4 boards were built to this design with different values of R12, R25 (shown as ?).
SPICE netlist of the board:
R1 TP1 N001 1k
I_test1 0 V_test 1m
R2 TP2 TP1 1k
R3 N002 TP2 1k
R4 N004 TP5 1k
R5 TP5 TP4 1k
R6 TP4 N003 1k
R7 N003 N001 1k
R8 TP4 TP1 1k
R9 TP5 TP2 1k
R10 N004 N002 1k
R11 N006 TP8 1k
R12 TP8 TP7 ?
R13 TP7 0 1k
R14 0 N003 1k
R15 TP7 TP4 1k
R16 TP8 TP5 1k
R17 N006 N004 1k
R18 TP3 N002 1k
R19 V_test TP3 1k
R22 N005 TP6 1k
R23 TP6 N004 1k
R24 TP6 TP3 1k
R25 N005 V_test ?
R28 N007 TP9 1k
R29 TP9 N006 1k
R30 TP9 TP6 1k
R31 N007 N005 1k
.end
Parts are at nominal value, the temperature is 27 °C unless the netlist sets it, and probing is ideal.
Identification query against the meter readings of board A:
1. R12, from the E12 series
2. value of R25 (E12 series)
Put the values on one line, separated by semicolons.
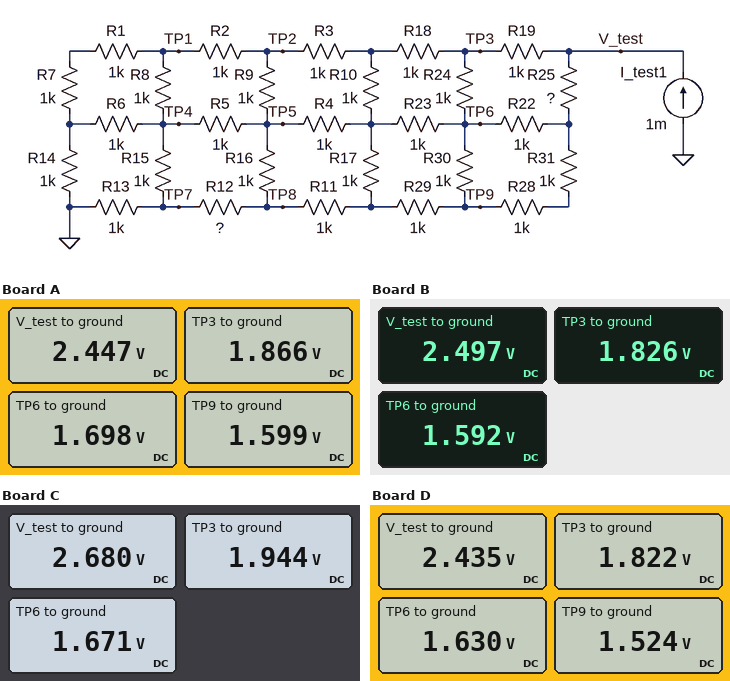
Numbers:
1.2 kΩ; 1.2 kΩ
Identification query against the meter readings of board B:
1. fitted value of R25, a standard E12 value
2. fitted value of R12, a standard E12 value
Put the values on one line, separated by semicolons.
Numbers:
2.2 kΩ; 680 Ω
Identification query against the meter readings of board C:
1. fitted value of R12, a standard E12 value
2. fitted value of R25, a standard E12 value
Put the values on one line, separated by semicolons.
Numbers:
1.2 kΩ; 3.3 kΩ
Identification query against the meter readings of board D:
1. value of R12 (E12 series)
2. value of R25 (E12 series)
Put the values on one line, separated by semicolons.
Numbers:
820 Ω; 1.5 kΩ
